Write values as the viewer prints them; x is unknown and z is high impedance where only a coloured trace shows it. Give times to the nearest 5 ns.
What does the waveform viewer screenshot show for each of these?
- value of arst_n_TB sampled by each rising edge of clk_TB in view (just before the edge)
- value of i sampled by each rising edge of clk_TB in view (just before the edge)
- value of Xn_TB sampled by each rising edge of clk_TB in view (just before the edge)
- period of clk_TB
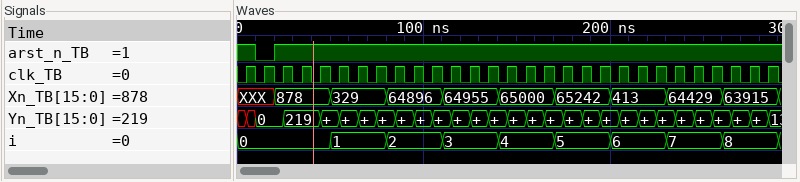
1 0 1 1 1 1 1 1 1 1 1 1 1 1 1 1 1 1 1 1 1 1 1 1 1 1 1 1 1
0, 0, 0, 0, 0, 1, 1, 1, 2, 2, 2, 3, 3, 3, 4, 4, 4, 5, 5, 5, 6, 6, 6, 7, 7, 7, 8, 8, 8
XXX, XXX, 878, 878, 878, 329, 329, 329, 64896, 64896, 64896, 64955, 64955, 64955, 65000, 65000, 65000, 65242, 65242, 65242, 413, 413, 413, 64429, 64429, 64429, 63915, 63915, 63915
10 ns
